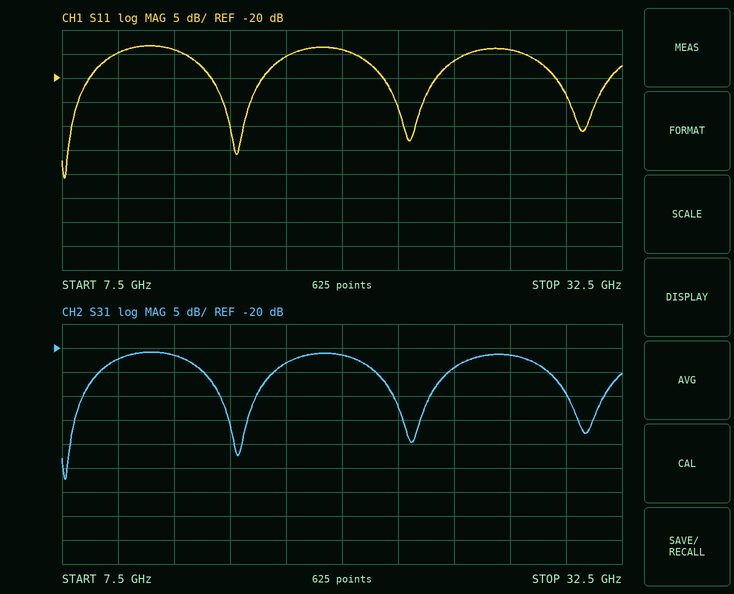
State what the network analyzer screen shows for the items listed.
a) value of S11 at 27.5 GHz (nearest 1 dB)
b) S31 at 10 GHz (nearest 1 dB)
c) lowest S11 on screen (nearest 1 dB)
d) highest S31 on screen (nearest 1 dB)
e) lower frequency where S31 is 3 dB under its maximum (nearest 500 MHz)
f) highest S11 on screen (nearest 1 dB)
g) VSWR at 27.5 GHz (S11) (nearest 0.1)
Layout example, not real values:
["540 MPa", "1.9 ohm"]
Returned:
["-14 dB", "-22 dB", "-41 dB", "-21 dB", "9.5 GHz", "-13 dB", "1.5"]
